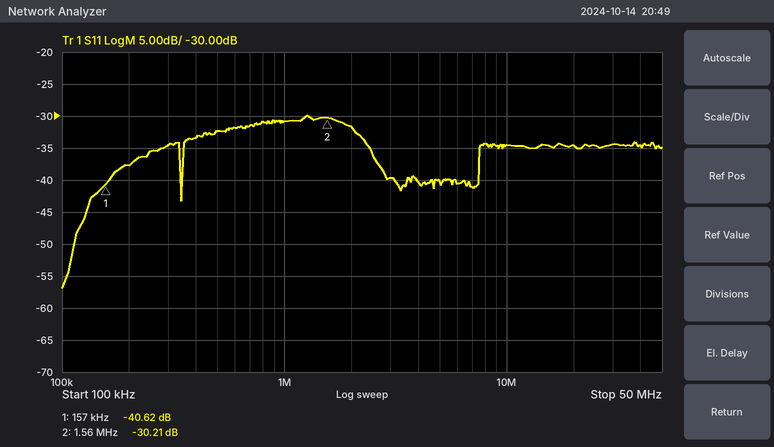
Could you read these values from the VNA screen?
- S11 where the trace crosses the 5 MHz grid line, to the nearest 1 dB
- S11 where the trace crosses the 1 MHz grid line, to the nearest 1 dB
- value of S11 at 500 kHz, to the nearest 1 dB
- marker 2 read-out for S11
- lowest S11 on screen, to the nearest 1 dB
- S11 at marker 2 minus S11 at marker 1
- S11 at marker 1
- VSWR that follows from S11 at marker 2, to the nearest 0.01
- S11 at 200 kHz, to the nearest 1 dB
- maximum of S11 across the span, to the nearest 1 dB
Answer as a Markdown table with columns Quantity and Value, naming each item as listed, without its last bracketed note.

| Quantity | Value |
|---|---|
| S11 where the trace crosses the 5 MHz grid line, to the nearest 1 dB | -40 dB |
| S11 where the trace crosses the 1 MHz grid line, to the nearest 1 dB | -31 dB |
| value of S11 at 500 kHz, to the nearest 1 dB | -32 dB |
| marker 2 read-out for S11 | -30.21 dB |
| lowest S11 on screen, to the nearest 1 dB | -57 dB |
| S11 at marker 2 minus S11 at marker 1 | 10.41 dB |
| S11 at marker 1 | -40.62 dB |
| VSWR that follows from S11 at marker 2, to the nearest 0.01 | 1.06 |
| S11 at 200 kHz, to the nearest 1 dB | -38 dB |
| maximum of S11 across the span, to the nearest 1 dB | -30 dB |
